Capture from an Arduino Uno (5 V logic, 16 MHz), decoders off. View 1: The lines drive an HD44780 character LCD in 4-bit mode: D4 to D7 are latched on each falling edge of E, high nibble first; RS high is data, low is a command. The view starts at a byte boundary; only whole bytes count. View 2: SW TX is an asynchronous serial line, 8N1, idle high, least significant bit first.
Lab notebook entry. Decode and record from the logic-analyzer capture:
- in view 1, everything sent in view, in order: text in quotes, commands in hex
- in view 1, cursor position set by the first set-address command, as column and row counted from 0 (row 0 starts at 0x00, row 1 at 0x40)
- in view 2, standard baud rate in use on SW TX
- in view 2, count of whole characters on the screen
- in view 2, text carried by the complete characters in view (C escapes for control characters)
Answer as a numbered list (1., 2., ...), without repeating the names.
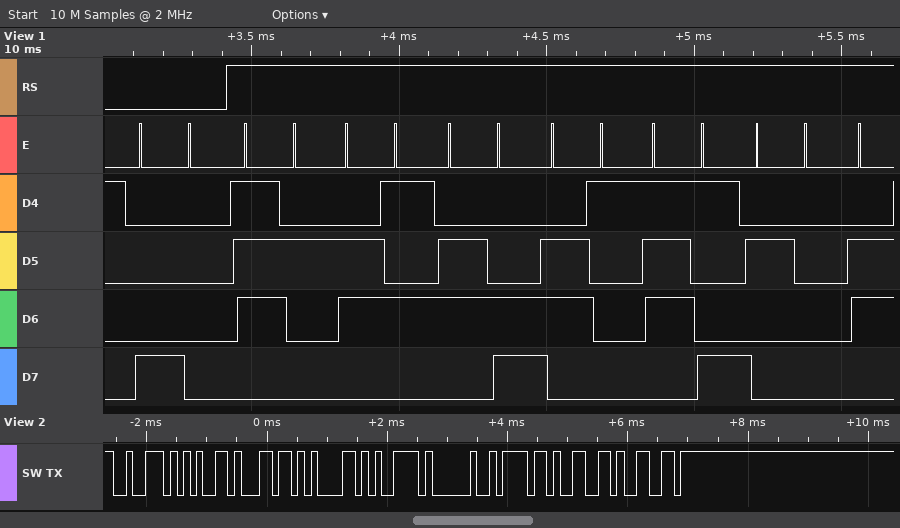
1. 0x80 "relay "
2. column 0, row 0
3. 9600 baud
4. 9
5. "relay off"
